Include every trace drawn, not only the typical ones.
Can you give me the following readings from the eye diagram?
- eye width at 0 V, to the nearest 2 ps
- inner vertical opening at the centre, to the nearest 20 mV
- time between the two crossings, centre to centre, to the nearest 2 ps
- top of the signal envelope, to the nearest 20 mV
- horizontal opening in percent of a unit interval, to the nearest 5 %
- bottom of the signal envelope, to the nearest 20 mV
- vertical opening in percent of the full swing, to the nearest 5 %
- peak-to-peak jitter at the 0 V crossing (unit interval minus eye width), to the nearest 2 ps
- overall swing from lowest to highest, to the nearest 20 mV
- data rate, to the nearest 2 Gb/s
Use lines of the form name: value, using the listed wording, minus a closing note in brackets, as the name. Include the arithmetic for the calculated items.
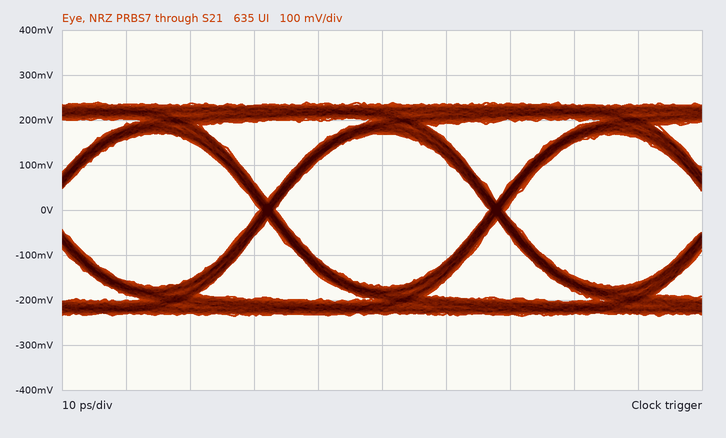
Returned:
eye width at 0 V, to the nearest 2 ps: 34 ps
inner vertical opening at the centre, to the nearest 20 mV: 340 mV
time between the two crossings, centre to centre, to the nearest 2 ps: 36 ps
top of the signal envelope, to the nearest 20 mV: 240 mV
horizontal opening in percent of a unit interval, to the nearest 5 %: 34 ps / 36 ps ≈ 94.4 %, so 95 % to the nearest 5 %
bottom of the signal envelope, to the nearest 20 mV: -240 mV
vertical opening in percent of the full swing, to the nearest 5 %: 340 mV / 480 mV ≈ 70.8 %, so 70 % to the nearest 5 %
peak-to-peak jitter at the 0 V crossing (unit interval minus eye width), to the nearest 2 ps: 2 ps
overall swing from lowest to highest, to the nearest 20 mV: 480 mV
data rate, to the nearest 2 Gb/s: 28 Gb/s
